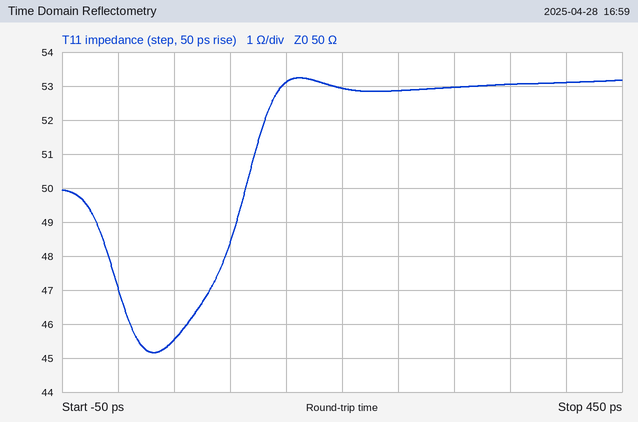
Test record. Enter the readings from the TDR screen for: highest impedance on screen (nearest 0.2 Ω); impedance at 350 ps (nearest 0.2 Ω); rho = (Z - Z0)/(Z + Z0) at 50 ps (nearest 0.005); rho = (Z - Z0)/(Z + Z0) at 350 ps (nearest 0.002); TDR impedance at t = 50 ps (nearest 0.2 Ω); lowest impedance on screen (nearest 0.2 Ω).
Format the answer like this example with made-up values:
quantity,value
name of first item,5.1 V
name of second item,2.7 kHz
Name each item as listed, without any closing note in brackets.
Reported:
quantity,value
highest impedance on screen,53.2 Ω
impedance at 350 ps,53.0 Ω
rho = (Z - Z0)/(Z + Z0) at 50 ps,-0.045
rho = (Z - Z0)/(Z + Z0) at 350 ps,+0.030
TDR impedance at t = 50 ps,45.6 Ω
lowest impedance on screen,45.2 Ω
